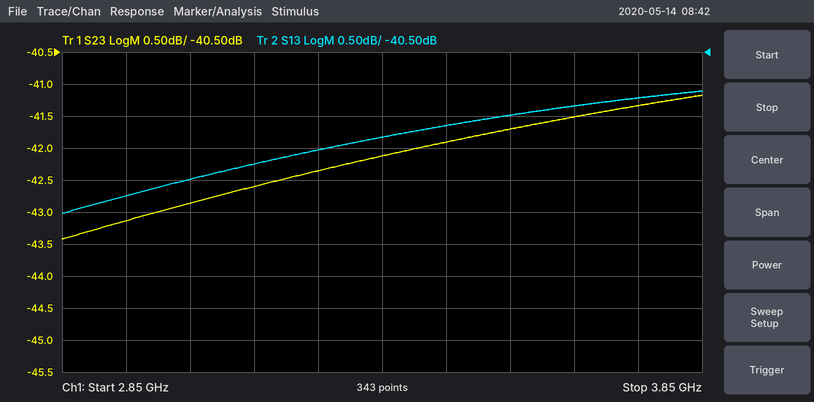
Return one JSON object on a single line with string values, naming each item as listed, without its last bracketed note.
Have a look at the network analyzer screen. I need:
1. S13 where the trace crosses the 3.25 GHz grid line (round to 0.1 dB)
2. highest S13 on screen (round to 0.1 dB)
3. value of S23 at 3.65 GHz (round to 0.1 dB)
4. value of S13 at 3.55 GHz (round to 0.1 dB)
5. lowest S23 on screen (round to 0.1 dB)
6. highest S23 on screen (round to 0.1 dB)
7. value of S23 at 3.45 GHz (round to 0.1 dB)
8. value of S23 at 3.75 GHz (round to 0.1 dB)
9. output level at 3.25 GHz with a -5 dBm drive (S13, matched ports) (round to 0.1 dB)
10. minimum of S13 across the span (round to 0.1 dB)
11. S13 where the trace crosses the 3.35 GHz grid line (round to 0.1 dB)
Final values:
{"S13 where the trace crosses the 3.25 GHz grid line": "-42.0 dB", "highest S13 on screen": "-41.1 dB", "value of S23 at 3.65 GHz": "-41.5 dB", "value of S13 at 3.55 GHz": "-41.5 dB", "lowest S23 on screen": "-43.4 dB", "highest S23 on screen": "-41.2 dB", "value of S23 at 3.45 GHz": "-41.9 dB", "value of S23 at 3.75 GHz": "-41.3 dB", "output level at 3.25 GHz with a -5 dBm drive (S13, matched ports)": "-47.0 dBm", "minimum of S13 across the span": "-43.0 dB", "S13 where the trace crosses the 3.35 GHz grid line": "-41.8 dB"}
